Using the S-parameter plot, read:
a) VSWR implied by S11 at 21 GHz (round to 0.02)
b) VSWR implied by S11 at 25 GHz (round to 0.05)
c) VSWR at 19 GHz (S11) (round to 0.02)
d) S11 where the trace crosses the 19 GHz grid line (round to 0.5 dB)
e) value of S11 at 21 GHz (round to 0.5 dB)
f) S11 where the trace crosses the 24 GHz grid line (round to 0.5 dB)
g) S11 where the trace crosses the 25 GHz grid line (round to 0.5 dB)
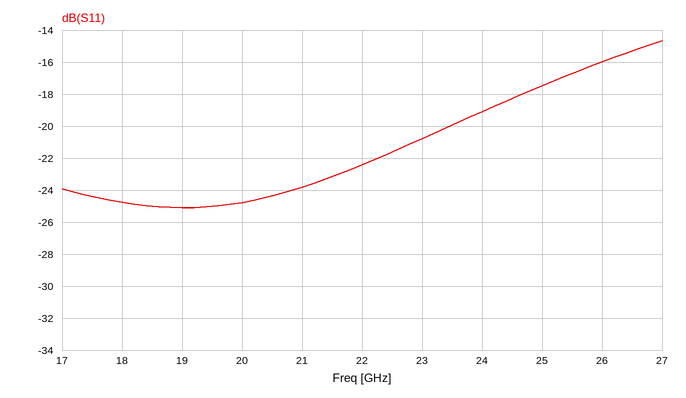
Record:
1.14
1.30
1.12
-25.0 dB
-24.0 dB
-19.0 dB
-17.5 dB
